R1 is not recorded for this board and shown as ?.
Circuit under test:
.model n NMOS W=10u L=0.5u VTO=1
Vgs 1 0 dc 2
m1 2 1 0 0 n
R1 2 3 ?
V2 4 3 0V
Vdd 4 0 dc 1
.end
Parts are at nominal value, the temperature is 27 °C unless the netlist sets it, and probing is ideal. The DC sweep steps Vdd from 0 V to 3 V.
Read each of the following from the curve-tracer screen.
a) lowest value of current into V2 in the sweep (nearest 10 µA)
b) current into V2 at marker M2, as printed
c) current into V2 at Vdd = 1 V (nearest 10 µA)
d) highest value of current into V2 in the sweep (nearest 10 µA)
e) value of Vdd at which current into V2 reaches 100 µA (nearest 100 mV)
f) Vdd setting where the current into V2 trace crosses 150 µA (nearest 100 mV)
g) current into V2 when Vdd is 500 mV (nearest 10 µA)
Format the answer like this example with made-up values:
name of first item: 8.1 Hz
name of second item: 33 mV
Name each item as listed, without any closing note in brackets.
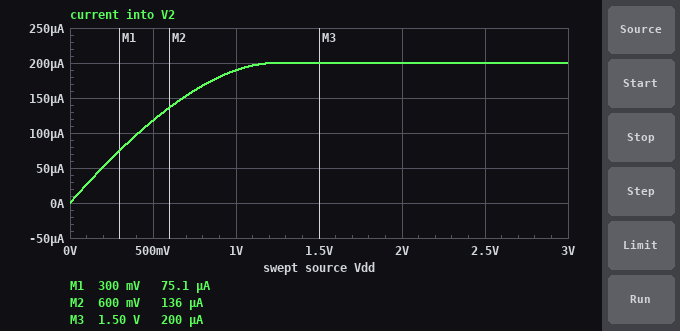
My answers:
lowest value of current into V2 in the sweep: 0 A
current into V2 at marker M2, as printed: 136 µA
current into V2 at Vdd = 1 V: 190 µA
highest value of current into V2 in the sweep: 200 µA
value of Vdd at which current into V2 reaches 100 µA: 400 mV
Vdd setting where the current into V2 trace crosses 150 µA: 700 mV
current into V2 when Vdd is 500 mV: 120 µA
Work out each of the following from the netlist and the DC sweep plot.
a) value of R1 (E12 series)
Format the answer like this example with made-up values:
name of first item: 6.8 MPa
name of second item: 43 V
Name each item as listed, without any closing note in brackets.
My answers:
value of R1: 1.2 kΩ
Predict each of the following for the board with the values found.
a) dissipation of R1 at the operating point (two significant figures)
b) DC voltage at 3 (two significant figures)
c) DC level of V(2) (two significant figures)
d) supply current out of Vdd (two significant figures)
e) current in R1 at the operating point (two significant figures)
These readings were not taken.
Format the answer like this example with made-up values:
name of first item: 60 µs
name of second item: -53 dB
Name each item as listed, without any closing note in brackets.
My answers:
dissipation of R1 at the operating point: 43 µW
DC voltage at 3: 1.0 V
DC level of V(2): 770 mV
supply current out of Vdd: 190 µA
current in R1 at the operating point: 190 µA
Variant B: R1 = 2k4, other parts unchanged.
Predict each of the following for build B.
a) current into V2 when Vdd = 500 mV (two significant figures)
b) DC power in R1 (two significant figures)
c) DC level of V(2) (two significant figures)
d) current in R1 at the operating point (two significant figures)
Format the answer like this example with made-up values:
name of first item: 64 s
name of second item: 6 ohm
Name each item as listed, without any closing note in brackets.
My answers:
current into V2 when Vdd = 500 mV: 94 µA
DC power in R1: 67 µW
DC level of V(2): 600 mV
current in R1 at the operating point: 170 µA
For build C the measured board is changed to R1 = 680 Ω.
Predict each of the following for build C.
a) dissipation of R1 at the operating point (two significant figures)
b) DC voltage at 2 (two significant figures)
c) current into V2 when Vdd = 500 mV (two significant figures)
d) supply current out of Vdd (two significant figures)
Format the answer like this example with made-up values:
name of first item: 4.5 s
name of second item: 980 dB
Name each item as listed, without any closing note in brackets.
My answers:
dissipation of R1 at the operating point: 26 µW
DC voltage at 2: 870 mV
current into V2 when Vdd = 500 mV: 130 µA
supply current out of Vdd: 200 µA
